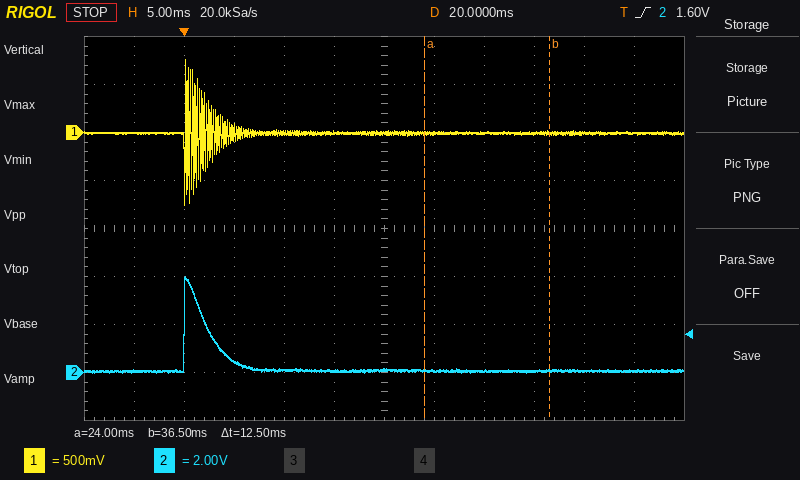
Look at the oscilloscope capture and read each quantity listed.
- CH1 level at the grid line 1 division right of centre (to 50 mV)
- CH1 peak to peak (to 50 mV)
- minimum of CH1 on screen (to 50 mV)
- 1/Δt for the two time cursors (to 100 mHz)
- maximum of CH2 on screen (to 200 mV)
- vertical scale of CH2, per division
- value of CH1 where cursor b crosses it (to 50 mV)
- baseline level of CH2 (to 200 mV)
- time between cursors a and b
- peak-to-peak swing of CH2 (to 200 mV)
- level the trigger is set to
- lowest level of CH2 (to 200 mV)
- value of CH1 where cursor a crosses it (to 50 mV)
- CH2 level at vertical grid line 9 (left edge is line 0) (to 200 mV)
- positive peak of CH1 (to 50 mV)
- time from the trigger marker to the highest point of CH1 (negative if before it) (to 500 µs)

0 mV
1.50 V
-750 mV
80.0 Hz
4.0 V
2 V
0 mV
0.0 V
12.5 ms
4.0 V
1.60 V
0.0 V
0 mV
0.0 V
750 mV
0.0 ms
